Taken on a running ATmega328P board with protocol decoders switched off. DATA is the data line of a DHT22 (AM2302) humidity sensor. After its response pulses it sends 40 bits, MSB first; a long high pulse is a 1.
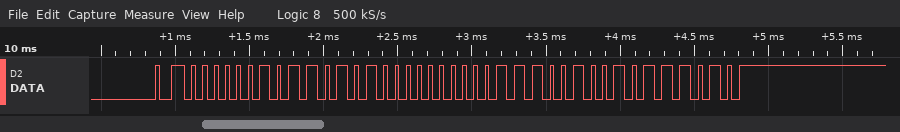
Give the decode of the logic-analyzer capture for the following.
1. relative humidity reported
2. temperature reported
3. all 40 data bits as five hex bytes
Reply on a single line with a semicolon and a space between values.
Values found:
72.4 %; 22.8 °C; 02 D4 00 E4 BA
